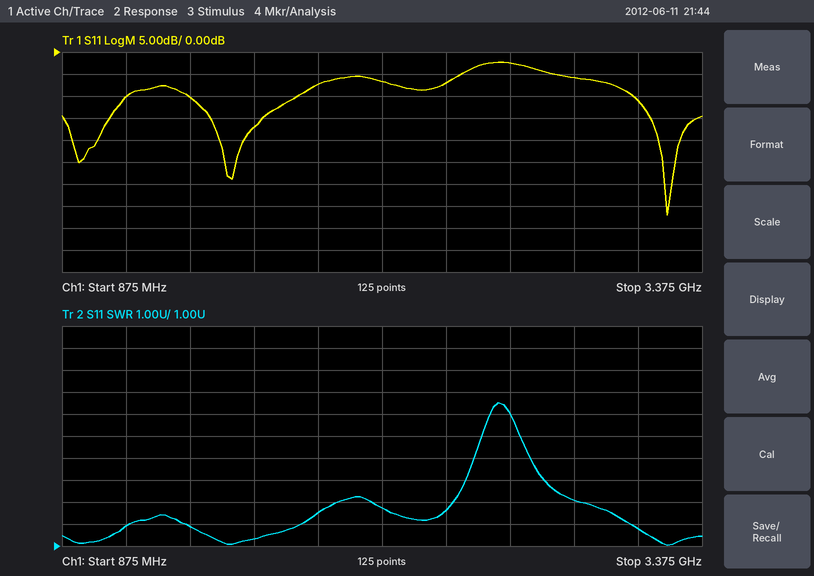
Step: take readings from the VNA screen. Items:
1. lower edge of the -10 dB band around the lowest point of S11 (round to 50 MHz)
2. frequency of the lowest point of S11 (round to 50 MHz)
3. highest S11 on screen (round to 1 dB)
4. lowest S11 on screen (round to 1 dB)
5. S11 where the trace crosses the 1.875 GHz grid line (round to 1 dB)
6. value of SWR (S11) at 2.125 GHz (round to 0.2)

3.10 GHz
3.25 GHz
-2 dB
-37 dB
-7 dB
2.8
